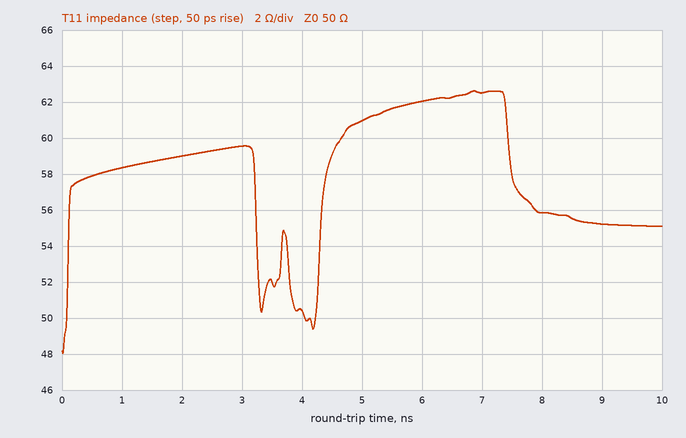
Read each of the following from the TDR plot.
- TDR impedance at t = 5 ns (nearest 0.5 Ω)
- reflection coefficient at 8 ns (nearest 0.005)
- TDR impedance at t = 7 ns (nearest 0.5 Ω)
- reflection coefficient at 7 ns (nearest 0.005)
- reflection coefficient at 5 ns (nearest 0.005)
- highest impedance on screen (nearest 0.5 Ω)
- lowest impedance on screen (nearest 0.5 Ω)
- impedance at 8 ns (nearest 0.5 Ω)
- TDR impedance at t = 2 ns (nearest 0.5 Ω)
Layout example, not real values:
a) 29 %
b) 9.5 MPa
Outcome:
a) 61.0 Ω
b) +0.055
c) 62.5 Ω
d) +0.110
e) +0.100
f) 62.5 Ω
g) 48.0 Ω
h) 56.0 Ω
i) 59.0 Ω
